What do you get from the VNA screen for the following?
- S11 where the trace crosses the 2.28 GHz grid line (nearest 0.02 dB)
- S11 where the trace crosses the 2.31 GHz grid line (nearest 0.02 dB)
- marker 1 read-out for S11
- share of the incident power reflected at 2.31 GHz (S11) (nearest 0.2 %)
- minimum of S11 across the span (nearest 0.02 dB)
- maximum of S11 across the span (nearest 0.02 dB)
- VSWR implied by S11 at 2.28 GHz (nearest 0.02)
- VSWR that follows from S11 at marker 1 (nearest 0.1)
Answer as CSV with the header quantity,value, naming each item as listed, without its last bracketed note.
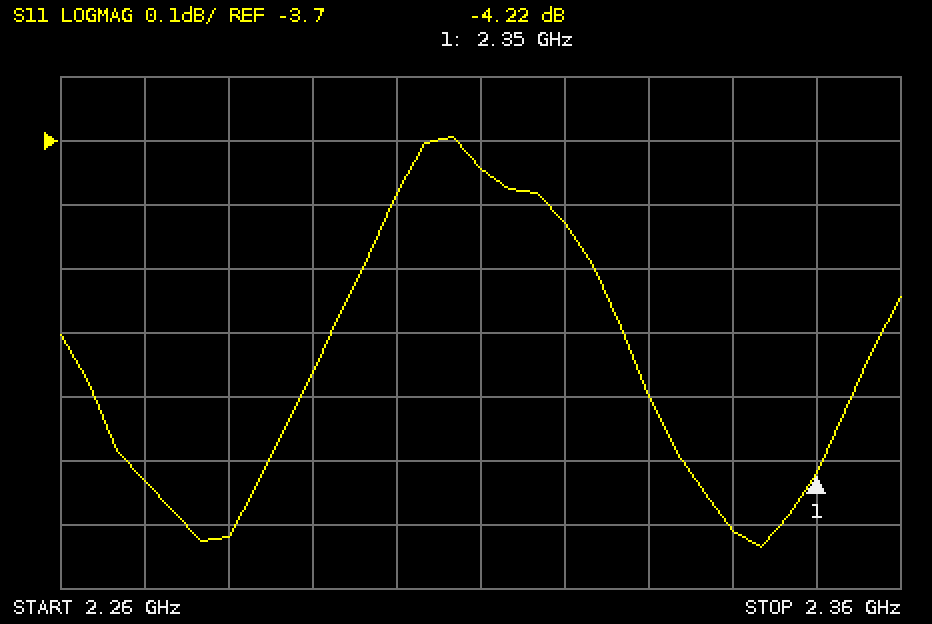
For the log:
quantity,value
S11 where the trace crosses the 2.28 GHz grid line,-4.32 dB
S11 where the trace crosses the 2.31 GHz grid line,-3.74 dB
marker 1 read-out for S11,-4.22 dB
share of the incident power reflected at 2.31 GHz (S11),42.2 %
minimum of S11 across the span,-4.34 dB
maximum of S11 across the span,-3.70 dB
VSWR implied by S11 at 2.28 GHz,4.10
VSWR that follows from S11 at marker 1,4.2
